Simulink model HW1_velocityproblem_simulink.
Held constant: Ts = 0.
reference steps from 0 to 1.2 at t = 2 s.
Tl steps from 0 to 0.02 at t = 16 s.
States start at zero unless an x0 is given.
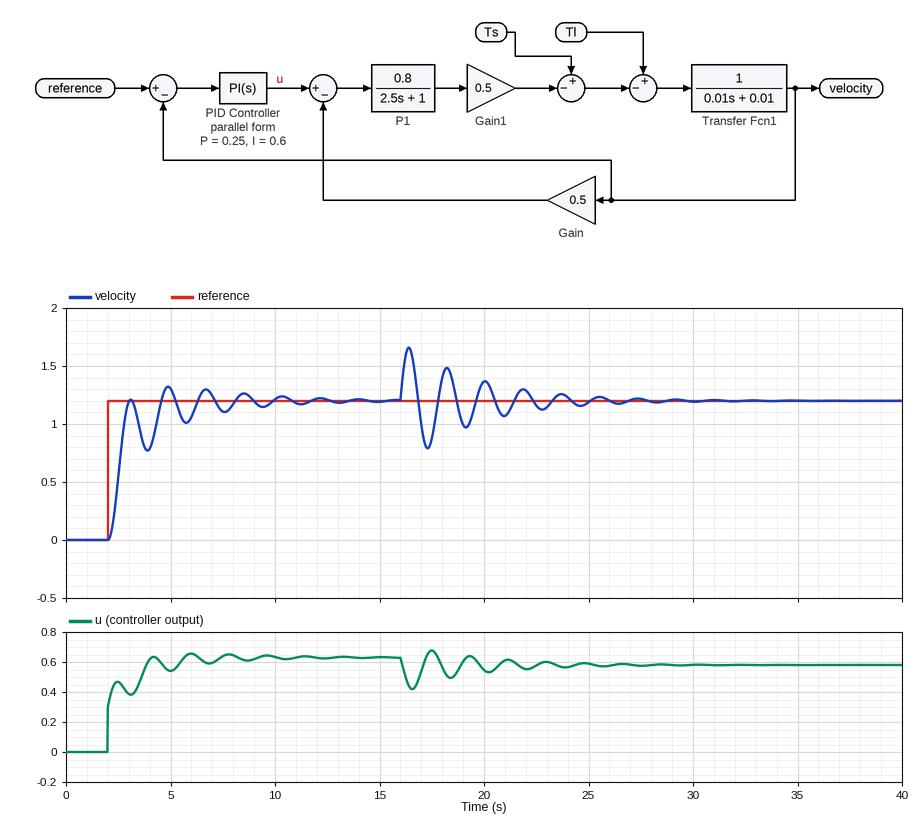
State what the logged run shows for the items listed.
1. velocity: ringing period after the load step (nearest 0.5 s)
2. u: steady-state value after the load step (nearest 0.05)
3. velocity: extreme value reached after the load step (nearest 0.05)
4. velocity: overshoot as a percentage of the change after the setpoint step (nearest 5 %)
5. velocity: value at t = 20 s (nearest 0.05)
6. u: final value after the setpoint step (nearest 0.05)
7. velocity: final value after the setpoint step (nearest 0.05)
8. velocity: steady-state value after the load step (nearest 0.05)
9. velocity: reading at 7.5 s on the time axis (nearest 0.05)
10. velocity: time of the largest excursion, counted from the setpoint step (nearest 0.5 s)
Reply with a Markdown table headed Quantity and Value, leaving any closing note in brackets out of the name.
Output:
| Quantity | Value |
|---|---|
| velocity: ringing period after the load step | 2.0 s |
| u: steady-state value after the load step | 0.60 |
| velocity: extreme value reached after the load step | 1.65 |
| velocity: overshoot as a percentage of the change after the setpoint step | 10 % |
| velocity: value at t = 20 s | 1.35 |
| u: final value after the setpoint step | 0.65 |
| velocity: final value after the setpoint step | 1.20 |
| velocity: steady-state value after the load step | 1.20 |
| velocity: reading at 7.5 s on the time axis | 1.10 |
| velocity: time of the largest excursion, counted from the setpoint step | 3.0 s |
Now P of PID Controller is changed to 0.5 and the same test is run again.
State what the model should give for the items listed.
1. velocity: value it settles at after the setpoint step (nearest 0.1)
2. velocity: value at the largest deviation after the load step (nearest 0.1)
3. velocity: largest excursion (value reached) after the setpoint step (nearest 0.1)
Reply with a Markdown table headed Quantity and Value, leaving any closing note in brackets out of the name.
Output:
| Quantity | Value |
|---|---|
| velocity: value it settles at after the setpoint step | 1.2 |
| velocity: value at the largest deviation after the load step | 1.6 |
| velocity: largest excursion (value reached) after the setpoint step | 1.3 |
